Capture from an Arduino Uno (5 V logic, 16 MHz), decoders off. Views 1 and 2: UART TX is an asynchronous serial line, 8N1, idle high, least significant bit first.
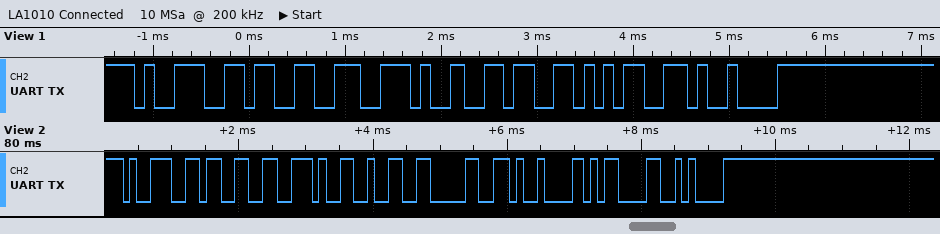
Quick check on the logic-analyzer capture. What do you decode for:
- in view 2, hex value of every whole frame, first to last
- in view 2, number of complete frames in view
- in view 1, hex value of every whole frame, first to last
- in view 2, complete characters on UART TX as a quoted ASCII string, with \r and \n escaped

39 33 2E 32 30 09 0D 0A
8
39 33 2E 36 35 09
"93.20\t\r\n"
